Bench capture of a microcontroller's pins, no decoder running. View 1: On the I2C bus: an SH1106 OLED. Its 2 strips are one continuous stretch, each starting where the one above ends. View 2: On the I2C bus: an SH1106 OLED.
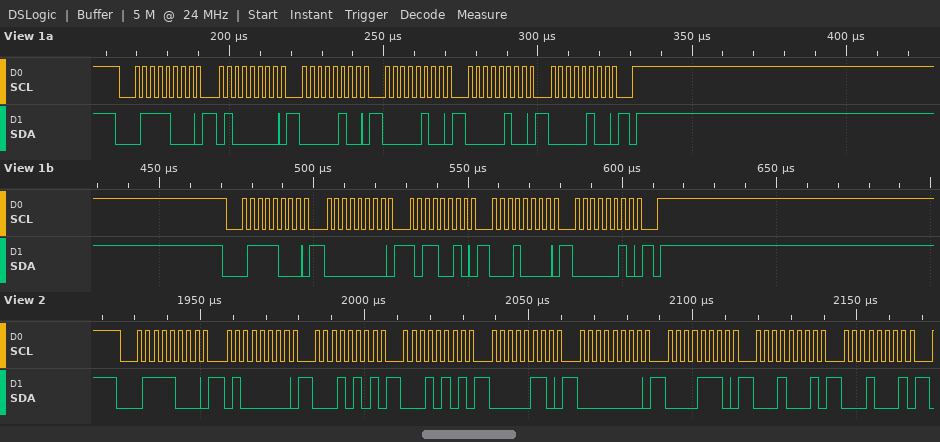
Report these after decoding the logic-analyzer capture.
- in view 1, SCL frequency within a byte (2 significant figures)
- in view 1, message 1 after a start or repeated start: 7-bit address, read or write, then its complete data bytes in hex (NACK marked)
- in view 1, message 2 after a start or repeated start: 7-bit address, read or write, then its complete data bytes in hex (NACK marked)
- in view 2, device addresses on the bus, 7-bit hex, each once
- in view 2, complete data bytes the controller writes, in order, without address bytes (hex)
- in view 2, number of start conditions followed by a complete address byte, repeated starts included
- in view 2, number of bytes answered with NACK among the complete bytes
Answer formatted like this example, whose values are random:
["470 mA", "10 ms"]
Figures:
["400 kHz", "0x3C write: 40 04 04 04 04", "0x3C write: 00 B2 10 02", "0x3C", "40 15 15 06 00 0E 11 11", "1", "0"]
